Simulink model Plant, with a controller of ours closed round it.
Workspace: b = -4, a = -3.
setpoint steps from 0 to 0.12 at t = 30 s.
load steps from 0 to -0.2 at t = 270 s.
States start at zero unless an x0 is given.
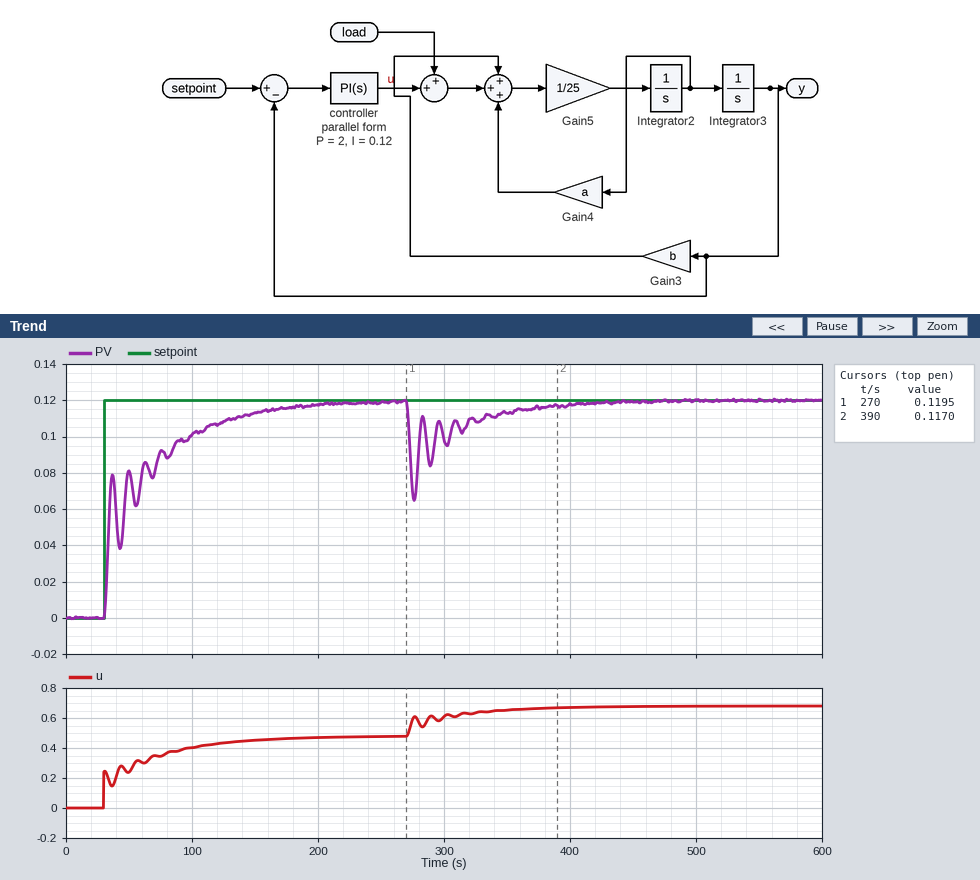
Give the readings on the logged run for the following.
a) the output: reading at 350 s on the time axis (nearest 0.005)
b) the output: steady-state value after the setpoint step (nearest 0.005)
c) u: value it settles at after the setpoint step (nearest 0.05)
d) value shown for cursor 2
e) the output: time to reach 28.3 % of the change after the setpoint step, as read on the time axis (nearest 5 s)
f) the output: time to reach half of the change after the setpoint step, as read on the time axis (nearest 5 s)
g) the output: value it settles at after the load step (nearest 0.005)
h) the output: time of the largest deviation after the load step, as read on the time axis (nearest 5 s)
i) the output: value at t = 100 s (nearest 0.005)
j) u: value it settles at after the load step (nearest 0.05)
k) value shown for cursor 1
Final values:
0.115
0.120
0.50
0.1170
35 s
35 s
0.120
275 s
0.100
0.70
0.1195
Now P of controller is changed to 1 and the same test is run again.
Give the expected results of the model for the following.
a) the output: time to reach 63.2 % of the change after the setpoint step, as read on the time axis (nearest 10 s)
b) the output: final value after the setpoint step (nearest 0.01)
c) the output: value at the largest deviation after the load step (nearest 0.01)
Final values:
60 s
0.12
0.06
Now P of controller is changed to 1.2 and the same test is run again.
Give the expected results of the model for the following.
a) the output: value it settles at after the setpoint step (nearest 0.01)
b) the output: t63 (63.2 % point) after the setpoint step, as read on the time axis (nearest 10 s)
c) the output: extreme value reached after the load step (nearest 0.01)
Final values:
0.12
60 s
0.06
